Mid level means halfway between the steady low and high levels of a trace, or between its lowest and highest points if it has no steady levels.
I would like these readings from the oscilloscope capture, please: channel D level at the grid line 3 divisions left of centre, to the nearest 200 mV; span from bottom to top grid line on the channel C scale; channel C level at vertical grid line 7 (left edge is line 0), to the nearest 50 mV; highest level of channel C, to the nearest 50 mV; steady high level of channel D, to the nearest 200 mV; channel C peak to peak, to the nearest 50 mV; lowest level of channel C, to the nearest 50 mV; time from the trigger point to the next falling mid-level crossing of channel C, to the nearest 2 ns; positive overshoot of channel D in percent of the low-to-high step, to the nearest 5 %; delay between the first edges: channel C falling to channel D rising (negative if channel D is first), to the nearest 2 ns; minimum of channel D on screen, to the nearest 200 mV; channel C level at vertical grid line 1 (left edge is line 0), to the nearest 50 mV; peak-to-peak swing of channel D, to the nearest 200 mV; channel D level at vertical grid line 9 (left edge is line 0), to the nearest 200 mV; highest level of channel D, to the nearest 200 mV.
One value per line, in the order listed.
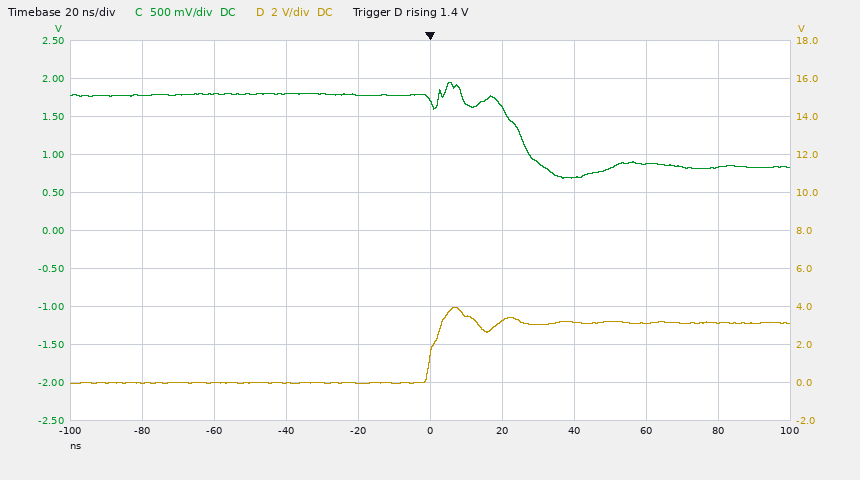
0.0 V
5 V
700 mV
1.95 V
3.2 V
1.25 V
700 mV
24 ns
25 %
-24 ns
0.0 V
1.80 V
4.0 V
3.2 V
4.0 V
